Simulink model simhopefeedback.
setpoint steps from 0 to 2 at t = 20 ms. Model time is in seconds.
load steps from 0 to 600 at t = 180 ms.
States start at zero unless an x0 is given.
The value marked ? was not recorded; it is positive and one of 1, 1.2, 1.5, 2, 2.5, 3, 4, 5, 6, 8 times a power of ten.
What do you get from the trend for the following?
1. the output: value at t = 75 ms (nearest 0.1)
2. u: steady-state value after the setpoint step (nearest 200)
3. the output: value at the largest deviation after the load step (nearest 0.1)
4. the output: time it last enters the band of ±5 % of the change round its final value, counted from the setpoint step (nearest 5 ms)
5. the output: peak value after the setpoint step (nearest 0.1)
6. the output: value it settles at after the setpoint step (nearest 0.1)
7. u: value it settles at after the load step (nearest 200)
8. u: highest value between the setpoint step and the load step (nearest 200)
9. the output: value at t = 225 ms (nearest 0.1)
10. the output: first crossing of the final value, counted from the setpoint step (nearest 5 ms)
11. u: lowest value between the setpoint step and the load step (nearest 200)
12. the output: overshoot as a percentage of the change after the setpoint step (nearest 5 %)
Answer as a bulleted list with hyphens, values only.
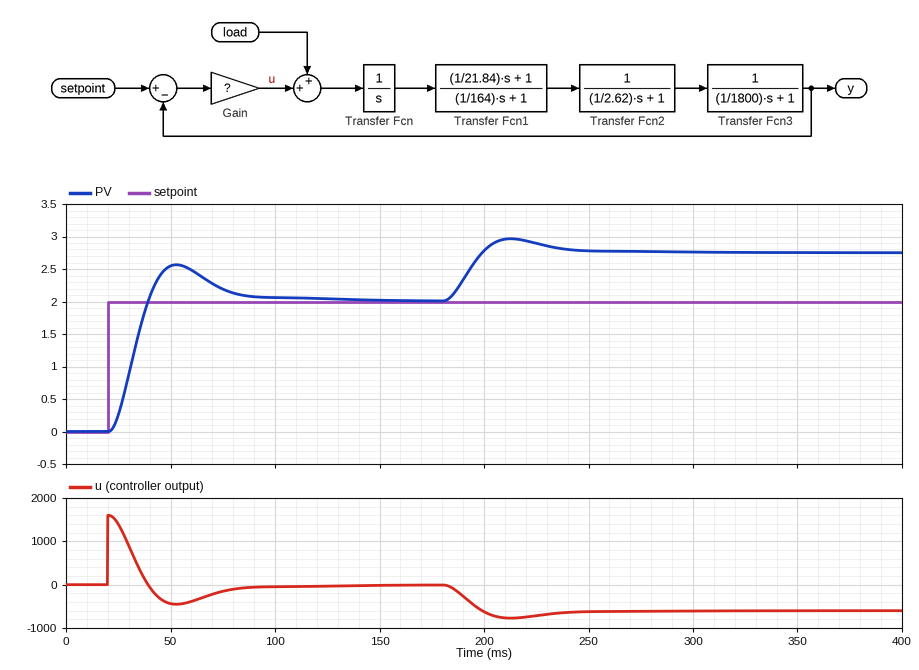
- 2.2
- 0
- 3.0
- 65 ms
- 2.6
- 2.0
- -600
- 1600
- 2.9
- 20 ms
- -400
- 30 %
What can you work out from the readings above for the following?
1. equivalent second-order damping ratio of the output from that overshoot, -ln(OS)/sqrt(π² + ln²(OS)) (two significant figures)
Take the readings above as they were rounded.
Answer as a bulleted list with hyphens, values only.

- 0.36
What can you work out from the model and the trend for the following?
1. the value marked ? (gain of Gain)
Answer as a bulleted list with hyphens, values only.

- 800
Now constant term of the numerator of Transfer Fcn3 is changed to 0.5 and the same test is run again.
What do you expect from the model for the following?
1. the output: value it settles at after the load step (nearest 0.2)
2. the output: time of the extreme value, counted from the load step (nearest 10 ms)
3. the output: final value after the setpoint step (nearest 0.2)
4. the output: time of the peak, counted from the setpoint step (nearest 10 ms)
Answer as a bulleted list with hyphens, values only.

- 2.8
- 60 ms
- 2.0
- 60 ms
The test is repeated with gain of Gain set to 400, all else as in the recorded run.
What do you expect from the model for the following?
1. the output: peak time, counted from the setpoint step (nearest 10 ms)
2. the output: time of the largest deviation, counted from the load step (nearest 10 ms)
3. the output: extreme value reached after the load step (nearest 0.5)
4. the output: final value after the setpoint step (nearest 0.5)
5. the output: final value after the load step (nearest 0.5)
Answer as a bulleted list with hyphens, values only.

- 60 ms
- 60 ms
- 4.0
- 2.0
- 3.5
